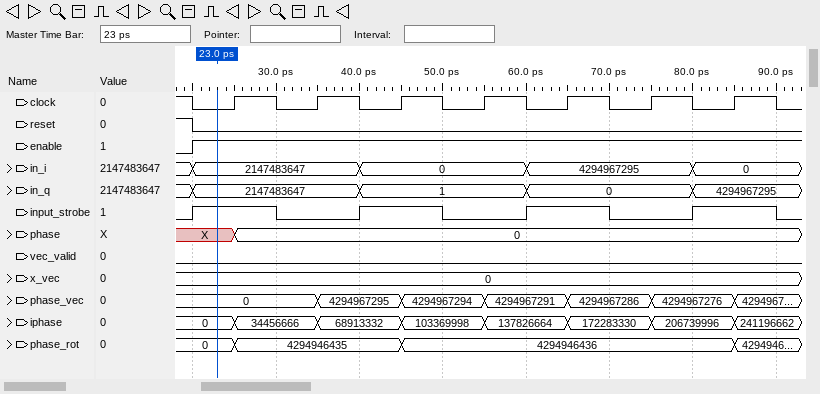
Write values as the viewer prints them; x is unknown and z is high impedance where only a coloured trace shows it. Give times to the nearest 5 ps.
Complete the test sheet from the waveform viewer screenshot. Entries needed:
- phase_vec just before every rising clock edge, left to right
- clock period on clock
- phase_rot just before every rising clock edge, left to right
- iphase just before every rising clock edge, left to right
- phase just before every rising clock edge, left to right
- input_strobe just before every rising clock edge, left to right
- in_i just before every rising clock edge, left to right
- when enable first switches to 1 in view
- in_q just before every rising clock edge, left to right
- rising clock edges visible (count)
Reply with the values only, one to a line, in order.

0, 0, 4294967295, 4294967294, 4294967291, 4294967286, 4294967276
10 ps
0, 4294946435, 4294946435, 4294946436, 4294946436, 4294946436, 4294946436
0, 34456666, 68913332, 103369998, 137826664, 172283330, 206739996
X, 0, 0, 0, 0, 0, 0
1 0 1 0 1 0 1
2147483647, 2147483647, 0, 0, 4294967295, 4294967295, 0
20 ps
2147483647, 2147483647, 1, 1, 0, 0, 4294967295
7
